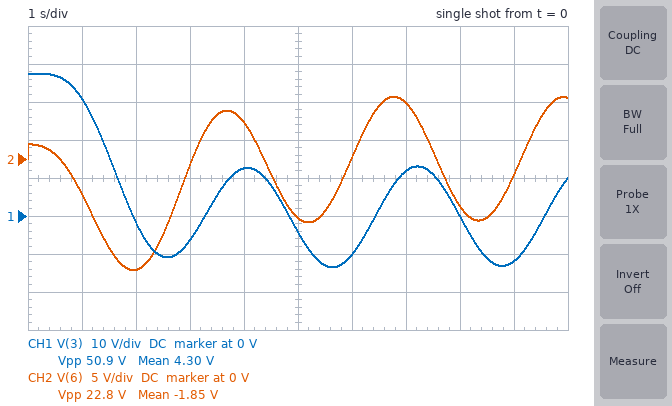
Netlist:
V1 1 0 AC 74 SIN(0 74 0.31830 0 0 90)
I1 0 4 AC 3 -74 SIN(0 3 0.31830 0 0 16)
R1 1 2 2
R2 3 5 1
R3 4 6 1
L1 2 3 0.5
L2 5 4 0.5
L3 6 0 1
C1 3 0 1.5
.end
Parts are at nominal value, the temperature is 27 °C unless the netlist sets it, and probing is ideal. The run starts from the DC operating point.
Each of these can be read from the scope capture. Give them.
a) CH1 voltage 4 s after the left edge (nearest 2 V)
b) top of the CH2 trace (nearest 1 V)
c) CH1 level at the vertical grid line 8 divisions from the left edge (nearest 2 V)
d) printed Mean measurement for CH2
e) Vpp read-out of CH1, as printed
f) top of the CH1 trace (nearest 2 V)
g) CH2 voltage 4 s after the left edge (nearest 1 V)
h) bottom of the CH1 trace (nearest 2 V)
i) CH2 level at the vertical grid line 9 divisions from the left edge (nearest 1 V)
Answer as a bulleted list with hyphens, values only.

- 12 V
- 8 V
- 0 V
- -1.85 V
- 50.9 V
- 38 V
- 5 V
- -14 V
- -2 V
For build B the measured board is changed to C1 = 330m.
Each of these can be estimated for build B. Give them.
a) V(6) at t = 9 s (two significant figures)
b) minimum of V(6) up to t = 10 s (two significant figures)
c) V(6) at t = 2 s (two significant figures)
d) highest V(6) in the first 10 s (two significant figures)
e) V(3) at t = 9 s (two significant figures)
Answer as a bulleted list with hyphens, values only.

- 15 V
- -34 V
- -26 V
- 34 V
- -9.8 V
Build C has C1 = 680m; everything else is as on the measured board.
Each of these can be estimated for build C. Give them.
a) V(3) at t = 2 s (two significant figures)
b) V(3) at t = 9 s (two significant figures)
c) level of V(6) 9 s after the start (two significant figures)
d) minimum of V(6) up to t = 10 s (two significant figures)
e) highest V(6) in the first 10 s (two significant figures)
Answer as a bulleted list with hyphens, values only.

- -31 V
- -23 V
- -2.2 V
- -24 V
- 20 V
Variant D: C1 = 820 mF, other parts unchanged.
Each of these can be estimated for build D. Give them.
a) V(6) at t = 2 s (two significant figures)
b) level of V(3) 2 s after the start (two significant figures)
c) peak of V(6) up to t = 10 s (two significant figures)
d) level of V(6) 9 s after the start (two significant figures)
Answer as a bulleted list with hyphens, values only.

- -21 V
- -24 V
- 16 V
- -3.0 V
